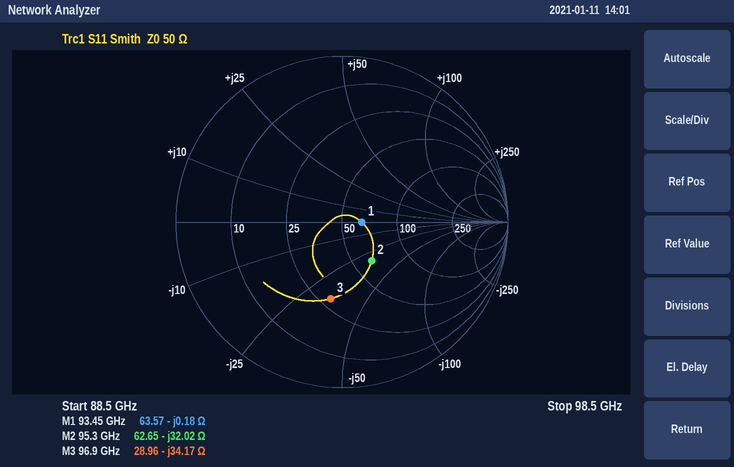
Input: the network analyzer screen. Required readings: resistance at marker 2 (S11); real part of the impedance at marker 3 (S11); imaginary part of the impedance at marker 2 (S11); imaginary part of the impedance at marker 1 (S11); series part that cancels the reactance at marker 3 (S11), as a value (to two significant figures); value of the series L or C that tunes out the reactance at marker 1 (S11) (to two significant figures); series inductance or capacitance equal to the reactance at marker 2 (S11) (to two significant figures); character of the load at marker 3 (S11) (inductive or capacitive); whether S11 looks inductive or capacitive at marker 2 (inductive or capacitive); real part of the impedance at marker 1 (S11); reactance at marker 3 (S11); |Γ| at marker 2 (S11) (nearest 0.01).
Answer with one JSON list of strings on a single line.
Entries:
["62.65 Ω", "28.96 Ω", "-32.02 Ω", "-0.18 Ω", "56 pH", "310 fH", "52 fF", "capacitive", "capacitive", "63.57 Ω", "-34.17 Ω", "0.29"]
